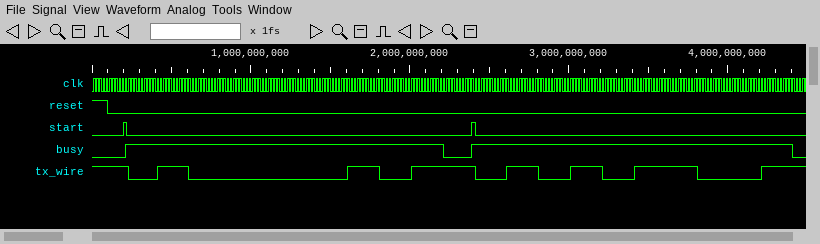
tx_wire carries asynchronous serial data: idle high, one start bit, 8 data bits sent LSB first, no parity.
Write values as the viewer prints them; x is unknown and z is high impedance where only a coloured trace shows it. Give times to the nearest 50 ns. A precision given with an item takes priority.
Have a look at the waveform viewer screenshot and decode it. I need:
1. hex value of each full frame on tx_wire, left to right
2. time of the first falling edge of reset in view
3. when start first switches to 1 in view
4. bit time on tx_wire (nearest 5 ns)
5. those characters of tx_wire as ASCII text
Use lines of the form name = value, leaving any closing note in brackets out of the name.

hex value of each full frame on tx_wire, left to right = 41, 35
time of the first falling edge of reset in view = 100 ns
when start first switches to 1 in view = 200 ns
bit time on tx_wire = 200 ns
those characters of tx_wire as ASCII text = "A5"
